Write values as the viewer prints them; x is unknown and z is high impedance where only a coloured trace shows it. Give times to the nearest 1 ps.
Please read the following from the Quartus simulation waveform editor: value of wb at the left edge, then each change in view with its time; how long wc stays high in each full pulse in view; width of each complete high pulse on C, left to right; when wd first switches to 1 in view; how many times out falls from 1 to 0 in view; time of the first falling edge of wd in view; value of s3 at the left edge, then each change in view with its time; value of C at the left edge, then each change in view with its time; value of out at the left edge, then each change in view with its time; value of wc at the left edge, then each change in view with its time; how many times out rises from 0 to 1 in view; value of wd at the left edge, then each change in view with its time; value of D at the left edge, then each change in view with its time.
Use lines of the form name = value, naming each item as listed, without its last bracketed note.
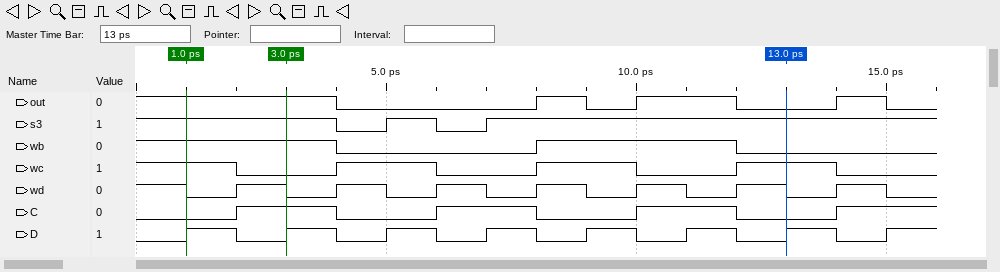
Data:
value of wb at the left edge, then each change in view with its time = 1, 0 at 4 ps, 1 at 8 ps, 0 at 12 ps
how long wc stays high in each full pulse in view = 2 ps, 2 ps, 2 ps
width of each complete high pulse on C, left to right = 2 ps, 2 ps, 2 ps
when wd first switches to 1 in view = 2 ps
how many times out falls from 1 to 0 in view = 4
time of the first falling edge of wd in view = 1 ps
value of s3 at the left edge, then each change in view with its time = 1, 0 at 4 ps, 1 at 5 ps, 0 at 6 ps, 1 at 7 ps
value of C at the left edge, then each change in view with its time = 0, 1 at 2 ps, 0 at 4 ps, 1 at 6 ps, 0 at 8 ps, 1 at 10 ps, 0 at 12 ps, 1 at 14 ps
value of out at the left edge, then each change in view with its time = 1, 0 at 4 ps, 1 at 8 ps, 0 at 9 ps, 1 at 10 ps, 0 at 12 ps, 1 at 14 ps, 0 at 15 ps
value of wc at the left edge, then each change in view with its time = 1, 0 at 2 ps, 1 at 4 ps, 0 at 6 ps, 1 at 8 ps, 0 at 10 ps, 1 at 12 ps, 0 at 14 ps
how many times out rises from 0 to 1 in view = 3
value of wd at the left edge, then each change in view with its time = 1, 0 at 1 ps, 1 at 2 ps, 0 at 3 ps, 1 at 4 ps, 0 at 5 ps, 1 at 6 ps, 0 at 7 ps, 1 at 8 ps, 0 at 9 ps, 1 at 10 ps, 0 at 11 ps, 1 at 12 ps, 0 at 13 ps, 1 at 14 ps, 0 at 15 ps
value of D at the left edge, then each change in view with its time = 0, 1 at 1 ps, 0 at 2 ps, 1 at 3 ps, 0 at 4 ps, 1 at 5 ps, 0 at 6 ps, 1 at 7 ps, 0 at 8 ps, 1 at 9 ps, 0 at 10 ps, 1 at 11 ps, 0 at 12 ps, 1 at 13 ps, 0 at 14 ps, 1 at 15 ps
